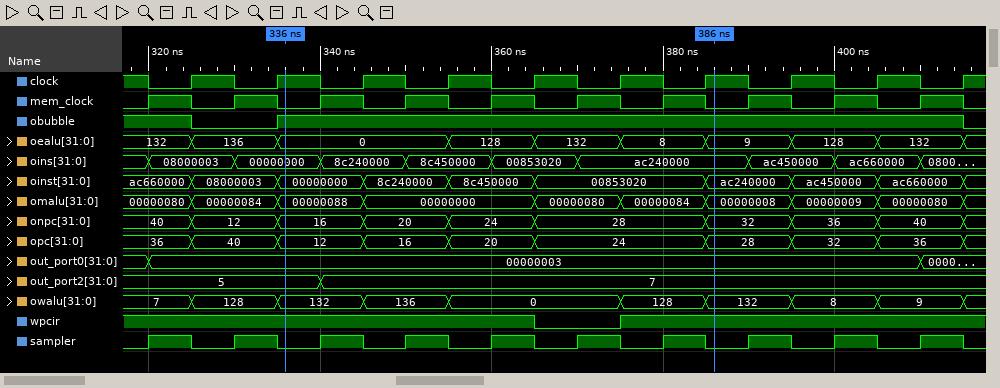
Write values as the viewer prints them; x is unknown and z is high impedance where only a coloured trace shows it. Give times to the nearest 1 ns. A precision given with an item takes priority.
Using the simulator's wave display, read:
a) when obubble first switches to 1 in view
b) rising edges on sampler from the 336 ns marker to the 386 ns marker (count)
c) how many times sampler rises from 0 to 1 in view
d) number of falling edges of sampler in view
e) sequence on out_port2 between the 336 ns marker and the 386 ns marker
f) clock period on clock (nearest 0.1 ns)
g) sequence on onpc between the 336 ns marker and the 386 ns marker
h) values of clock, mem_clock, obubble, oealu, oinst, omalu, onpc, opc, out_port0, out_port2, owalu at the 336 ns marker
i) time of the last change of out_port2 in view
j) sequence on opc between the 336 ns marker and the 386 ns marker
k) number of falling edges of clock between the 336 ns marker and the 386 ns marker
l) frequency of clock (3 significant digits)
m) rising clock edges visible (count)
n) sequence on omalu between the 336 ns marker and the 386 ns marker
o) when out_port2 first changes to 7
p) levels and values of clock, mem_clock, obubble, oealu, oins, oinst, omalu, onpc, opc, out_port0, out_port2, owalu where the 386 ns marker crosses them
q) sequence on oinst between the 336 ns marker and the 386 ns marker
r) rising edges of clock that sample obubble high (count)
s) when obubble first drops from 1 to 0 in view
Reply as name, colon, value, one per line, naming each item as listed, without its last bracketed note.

when obubble first switches to 1 in view: 335 ns
rising edges on sampler from the 336 ns marker to the 386 ns marker: 5
how many times sampler rises from 0 to 1 in view: 10
number of falling edges of sampler in view: 10
sequence on out_port2 between the 336 ns marker and the 386 ns marker: 5, 7
clock period on clock: 10 ns
sequence on onpc between the 336 ns marker and the 386 ns marker: 16, 20, 24, 28, 32
values of clock, mem_clock, obubble, oealu, oinst, omalu, onpc, opc, out_port0, out_port2, owalu at the 336 ns marker: clock=1, mem_clock=0, obubble=1, oealu=0, oinst=00000000, omalu=00000088, onpc=16, opc=12, out_port0=00000003, out_port2=5, owalu=132
time of the last change of out_port2 in view: 340 ns
sequence on opc between the 336 ns marker and the 386 ns marker: 12, 16, 20, 24, 28
number of falling edges of clock between the 336 ns marker and the 386 ns marker: 5
frequency of clock: 100 MHz
rising clock edges visible: 10
sequence on omalu between the 336 ns marker and the 386 ns marker: 00000088, 00000000, 00000080, 00000084, 00000008
when out_port2 first changes to 7: 340 ns
levels and values of clock, mem_clock, obubble, oealu, oins, oinst, omalu, onpc, opc, out_port0, out_port2, owalu where the 386 ns marker crosses them: clock=1, mem_clock=0, obubble=1, oealu=9, oins=ac240000, oinst=ac240000, omalu=00000008, onpc=32, opc=28, out_port0=00000003, out_port2=7, owalu=132
sequence on oinst between the 336 ns marker and the 386 ns marker: 00000000, 8c240000, 8c450000, 00853020, ac240000
rising edges of clock that sample obubble high: 9
when obubble first drops from 1 to 0 in view: 325 ns
